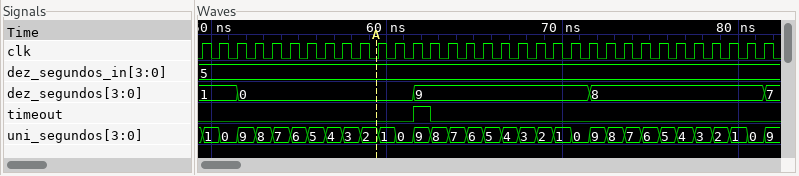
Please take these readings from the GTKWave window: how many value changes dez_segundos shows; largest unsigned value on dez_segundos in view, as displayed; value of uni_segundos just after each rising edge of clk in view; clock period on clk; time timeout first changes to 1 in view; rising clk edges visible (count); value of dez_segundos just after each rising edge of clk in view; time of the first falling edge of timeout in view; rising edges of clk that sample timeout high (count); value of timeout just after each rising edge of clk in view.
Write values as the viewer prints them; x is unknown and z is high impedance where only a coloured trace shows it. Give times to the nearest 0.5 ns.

4
9
1, 0, 9, 8, 7, 6, 5, 4, 3, 2, 1, 0, 9, 8, 7, 6, 5, 4, 3, 2, 1, 0, 9, 8, 7, 6, 5, 4, 3, 2, 1, 0, 9
1 ns
61.5 ns
33
1, 1, 0, 0, 0, 0, 0, 0, 0, 0, 0, 0, 9, 9, 9, 9, 9, 9, 9, 9, 9, 9, 8, 8, 8, 8, 8, 8, 8, 8, 8, 8, 7
62.5 ns
1
0 0 0 0 0 0 0 0 0 0 0 0 1 0 0 0 0 0 0 0 0 0 0 0 0 0 0 0 0 0 0 0 0
